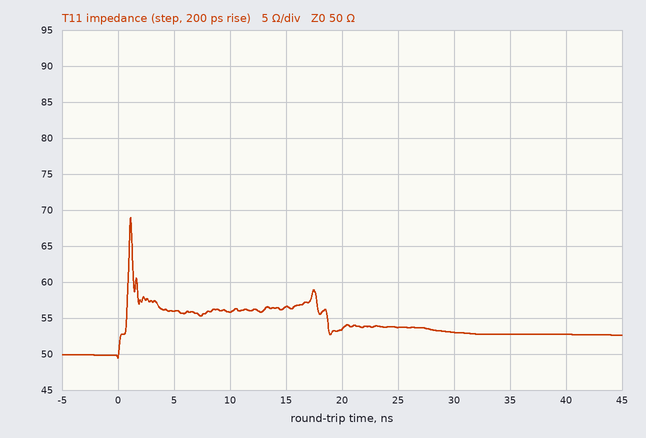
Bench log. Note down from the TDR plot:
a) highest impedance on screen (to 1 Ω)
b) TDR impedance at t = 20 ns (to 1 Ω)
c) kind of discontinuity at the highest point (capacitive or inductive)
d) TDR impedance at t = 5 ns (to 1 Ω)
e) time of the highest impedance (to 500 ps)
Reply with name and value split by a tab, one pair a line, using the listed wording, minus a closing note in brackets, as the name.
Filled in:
highest impedance on screen	69 Ω
TDR impedance at t = 20 ns	53 Ω
kind of discontinuity at the highest point	inductive
TDR impedance at t = 5 ns	56 Ω
time of the highest impedance	1.0 ns
